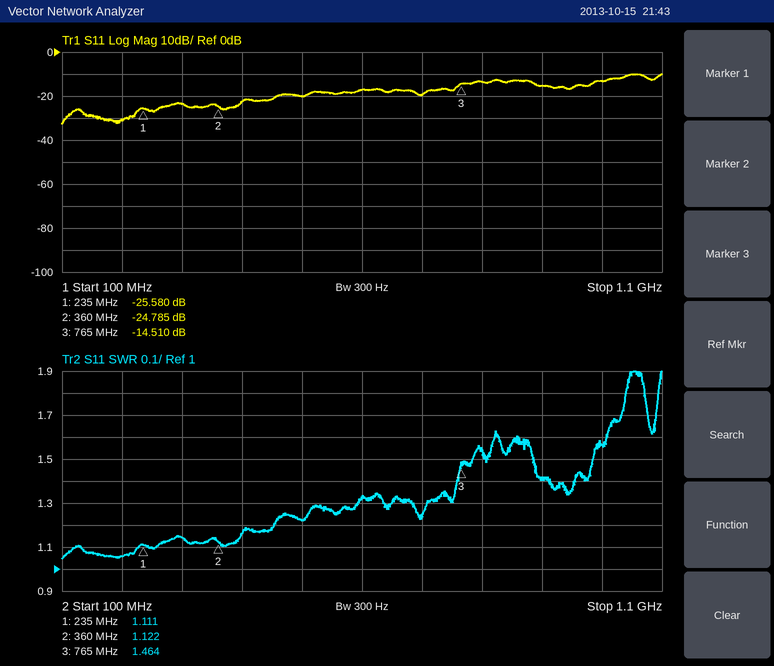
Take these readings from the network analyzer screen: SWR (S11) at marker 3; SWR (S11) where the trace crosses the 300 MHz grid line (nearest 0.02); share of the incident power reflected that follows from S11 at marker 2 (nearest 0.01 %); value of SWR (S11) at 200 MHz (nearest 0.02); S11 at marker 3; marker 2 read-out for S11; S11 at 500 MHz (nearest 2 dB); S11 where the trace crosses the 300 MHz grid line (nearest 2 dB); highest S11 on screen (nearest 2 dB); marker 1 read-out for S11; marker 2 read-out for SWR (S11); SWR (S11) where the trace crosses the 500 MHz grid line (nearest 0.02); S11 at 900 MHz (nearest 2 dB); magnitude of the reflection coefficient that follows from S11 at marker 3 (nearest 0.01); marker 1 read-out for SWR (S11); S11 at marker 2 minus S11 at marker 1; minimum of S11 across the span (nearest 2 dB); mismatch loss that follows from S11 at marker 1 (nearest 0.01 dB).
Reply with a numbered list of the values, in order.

1. 1.464
2. 1.14
3. 0.33 %
4. 1.06
5. -14.510 dB
6. -24.785 dB
7. -20 dB
8. -24 dB
9. -10 dB
10. -25.580 dB
11. 1.122
12. 1.22
13. -16 dB
14. 0.19
15. 1.111
16. 0.795 dB
17. -32 dB
18. 0.01 dB
